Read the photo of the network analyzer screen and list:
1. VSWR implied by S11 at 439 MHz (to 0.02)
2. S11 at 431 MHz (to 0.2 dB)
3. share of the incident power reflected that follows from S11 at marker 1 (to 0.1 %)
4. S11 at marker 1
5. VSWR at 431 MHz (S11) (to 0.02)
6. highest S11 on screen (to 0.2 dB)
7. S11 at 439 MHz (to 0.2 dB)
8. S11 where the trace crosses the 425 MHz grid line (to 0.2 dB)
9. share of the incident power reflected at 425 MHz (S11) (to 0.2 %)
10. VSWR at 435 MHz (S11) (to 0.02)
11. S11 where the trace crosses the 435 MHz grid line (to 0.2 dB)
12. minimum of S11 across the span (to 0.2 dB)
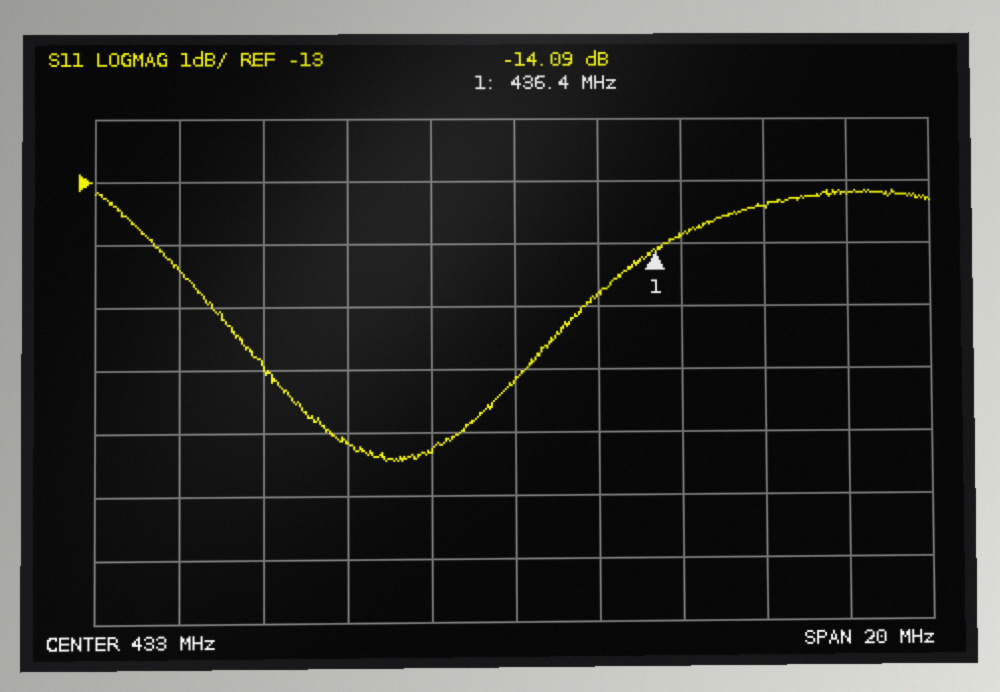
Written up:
1.54
-17.2 dB
3.9 %
-14.09 dB
1.32
-13.2 dB
-13.4 dB
-14.4 dB
3.6 %
1.44
-14.8 dB
-17.4 dB
